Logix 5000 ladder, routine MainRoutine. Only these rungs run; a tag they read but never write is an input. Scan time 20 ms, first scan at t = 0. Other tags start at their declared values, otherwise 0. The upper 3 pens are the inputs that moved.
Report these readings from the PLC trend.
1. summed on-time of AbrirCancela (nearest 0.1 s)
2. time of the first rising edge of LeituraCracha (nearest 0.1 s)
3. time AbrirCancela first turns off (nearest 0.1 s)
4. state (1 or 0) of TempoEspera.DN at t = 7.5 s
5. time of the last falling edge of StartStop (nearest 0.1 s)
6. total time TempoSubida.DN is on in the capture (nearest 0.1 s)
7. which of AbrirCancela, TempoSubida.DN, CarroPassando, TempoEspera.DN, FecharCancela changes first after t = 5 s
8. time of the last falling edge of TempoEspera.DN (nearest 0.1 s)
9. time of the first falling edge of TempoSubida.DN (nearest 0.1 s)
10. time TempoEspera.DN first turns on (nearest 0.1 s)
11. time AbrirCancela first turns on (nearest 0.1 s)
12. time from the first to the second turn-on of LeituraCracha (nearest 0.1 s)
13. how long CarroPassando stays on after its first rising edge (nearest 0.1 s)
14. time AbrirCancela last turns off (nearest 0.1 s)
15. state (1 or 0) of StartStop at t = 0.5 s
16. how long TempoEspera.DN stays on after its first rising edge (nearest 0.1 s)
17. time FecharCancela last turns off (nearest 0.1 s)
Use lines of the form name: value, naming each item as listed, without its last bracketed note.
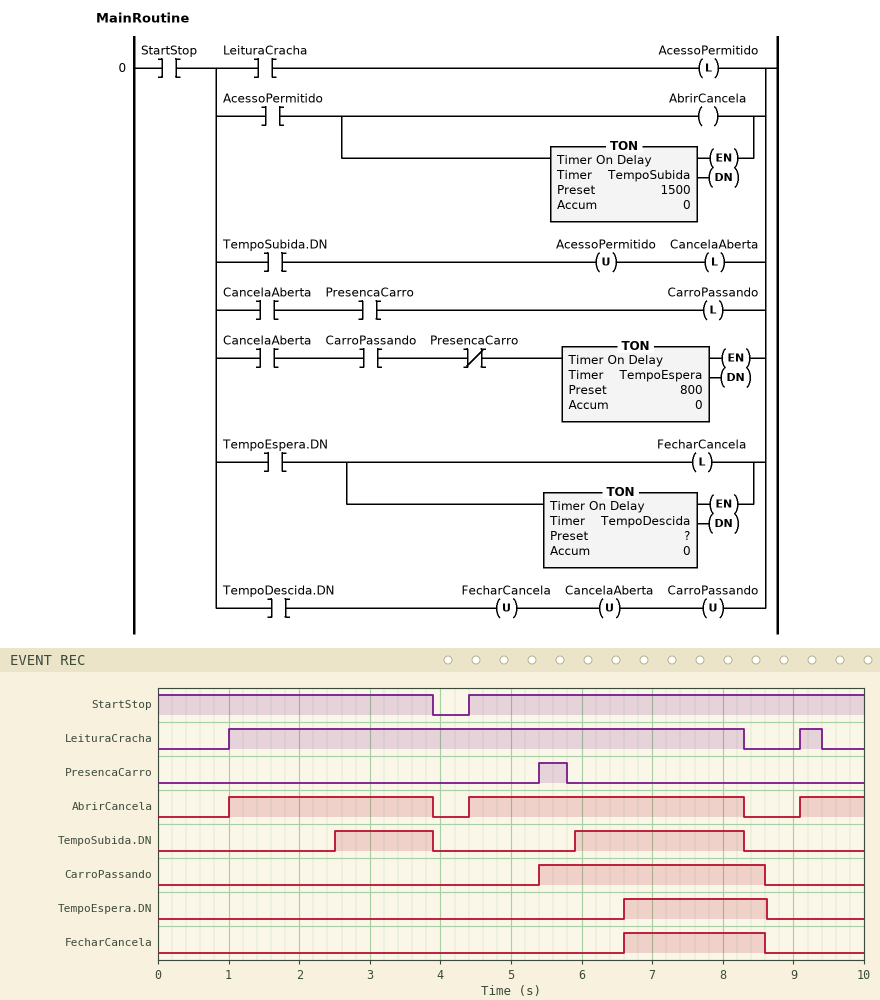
summed on-time of AbrirCancela: 7.7 s
time of the first rising edge of LeituraCracha: 1.0 s
time AbrirCancela first turns off: 3.9 s
state (1 or 0) of TempoEspera.DN at t = 7.5 s: 1
time of the last falling edge of StartStop: 3.9 s
total time TempoSubida.DN is on in the capture: 3.8 s
which of AbrirCancela, TempoSubida.DN, CarroPassando, TempoEspera.DN, FecharCancela changes first after t = 5 s: CarroPassando
time of the last falling edge of TempoEspera.DN: 8.6 s
time of the first falling edge of TempoSubida.DN: 3.9 s
time TempoEspera.DN first turns on: 6.6 s
time AbrirCancela first turns on: 1.0 s
time from the first to the second turn-on of LeituraCracha: 8.1 s
how long CarroPassando stays on after its first rising edge: 3.2 s
time AbrirCancela last turns off: 8.3 s
state (1 or 0) of StartStop at t = 0.5 s: 1
how long TempoEspera.DN stays on after its first rising edge: 2.0 s
time FecharCancela last turns off: 8.6 s
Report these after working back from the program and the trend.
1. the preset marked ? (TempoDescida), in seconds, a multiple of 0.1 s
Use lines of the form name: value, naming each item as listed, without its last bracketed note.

the preset marked ? (TempoDescida), in seconds, a multiple of 0.1 s: 2.0 s
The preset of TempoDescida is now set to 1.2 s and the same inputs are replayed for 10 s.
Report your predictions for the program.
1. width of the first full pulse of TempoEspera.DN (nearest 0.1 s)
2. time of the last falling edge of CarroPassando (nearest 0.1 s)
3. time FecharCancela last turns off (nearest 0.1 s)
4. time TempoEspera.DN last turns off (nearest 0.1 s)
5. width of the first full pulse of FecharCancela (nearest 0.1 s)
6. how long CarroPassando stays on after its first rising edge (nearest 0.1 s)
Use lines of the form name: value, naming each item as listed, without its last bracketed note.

width of the first full pulse of TempoEspera.DN: 1.2 s
time of the last falling edge of CarroPassando: 7.8 s
time FecharCancela last turns off: 7.8 s
time TempoEspera.DN last turns off: 7.8 s
width of the first full pulse of FecharCancela: 1.2 s
how long CarroPassando stays on after its first rising edge: 2.4 s
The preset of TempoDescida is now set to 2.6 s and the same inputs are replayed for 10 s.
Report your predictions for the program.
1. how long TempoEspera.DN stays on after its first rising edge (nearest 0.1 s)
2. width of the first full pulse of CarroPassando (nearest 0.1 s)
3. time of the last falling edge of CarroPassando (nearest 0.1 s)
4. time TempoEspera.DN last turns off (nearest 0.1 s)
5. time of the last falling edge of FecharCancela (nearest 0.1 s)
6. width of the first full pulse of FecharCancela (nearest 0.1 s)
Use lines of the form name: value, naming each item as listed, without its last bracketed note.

how long TempoEspera.DN stays on after its first rising edge: 2.6 s
width of the first full pulse of CarroPassando: 3.8 s
time of the last falling edge of CarroPassando: 9.2 s
time TempoEspera.DN last turns off: 9.2 s
time of the last falling edge of FecharCancela: 9.2 s
width of the first full pulse of FecharCancela: 2.6 s
